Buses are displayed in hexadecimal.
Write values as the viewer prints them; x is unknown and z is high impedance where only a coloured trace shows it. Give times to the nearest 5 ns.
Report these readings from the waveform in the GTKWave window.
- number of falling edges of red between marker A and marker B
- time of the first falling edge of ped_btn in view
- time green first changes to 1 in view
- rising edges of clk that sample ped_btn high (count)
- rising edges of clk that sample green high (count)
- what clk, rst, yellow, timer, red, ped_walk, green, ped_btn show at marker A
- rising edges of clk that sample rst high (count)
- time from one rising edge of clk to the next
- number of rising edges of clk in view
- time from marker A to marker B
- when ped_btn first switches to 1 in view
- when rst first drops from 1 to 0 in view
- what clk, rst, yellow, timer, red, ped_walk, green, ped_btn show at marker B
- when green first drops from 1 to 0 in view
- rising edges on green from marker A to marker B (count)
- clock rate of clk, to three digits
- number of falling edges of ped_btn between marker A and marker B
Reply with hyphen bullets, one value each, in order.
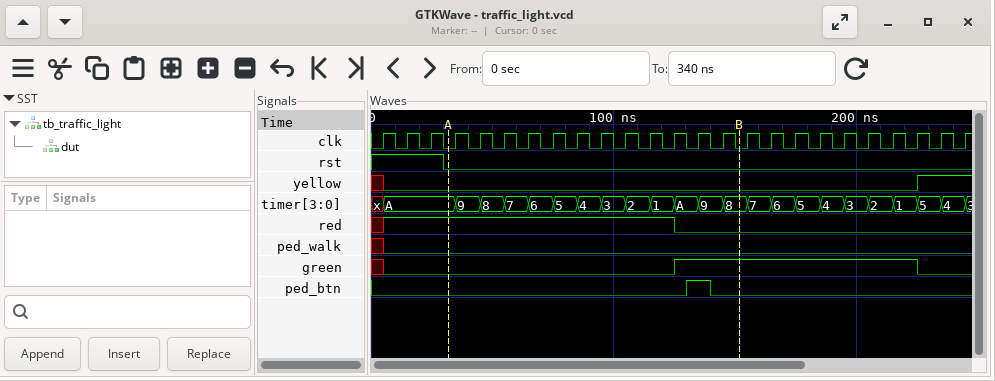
- 1
- 140 ns
- 125 ns
- 1
- 10
- clk=0, rst=0, yellow=0, timer=A, red=1, ped_walk=0, green=0, ped_btn=0
- 3
- 10 ns
- 25
- 120 ns
- 130 ns
- 30 ns
- clk=0, rst=0, yellow=0, timer=8, red=0, ped_walk=0, green=1, ped_btn=0
- 225 ns
- 1
- 100 MHz
- 1
